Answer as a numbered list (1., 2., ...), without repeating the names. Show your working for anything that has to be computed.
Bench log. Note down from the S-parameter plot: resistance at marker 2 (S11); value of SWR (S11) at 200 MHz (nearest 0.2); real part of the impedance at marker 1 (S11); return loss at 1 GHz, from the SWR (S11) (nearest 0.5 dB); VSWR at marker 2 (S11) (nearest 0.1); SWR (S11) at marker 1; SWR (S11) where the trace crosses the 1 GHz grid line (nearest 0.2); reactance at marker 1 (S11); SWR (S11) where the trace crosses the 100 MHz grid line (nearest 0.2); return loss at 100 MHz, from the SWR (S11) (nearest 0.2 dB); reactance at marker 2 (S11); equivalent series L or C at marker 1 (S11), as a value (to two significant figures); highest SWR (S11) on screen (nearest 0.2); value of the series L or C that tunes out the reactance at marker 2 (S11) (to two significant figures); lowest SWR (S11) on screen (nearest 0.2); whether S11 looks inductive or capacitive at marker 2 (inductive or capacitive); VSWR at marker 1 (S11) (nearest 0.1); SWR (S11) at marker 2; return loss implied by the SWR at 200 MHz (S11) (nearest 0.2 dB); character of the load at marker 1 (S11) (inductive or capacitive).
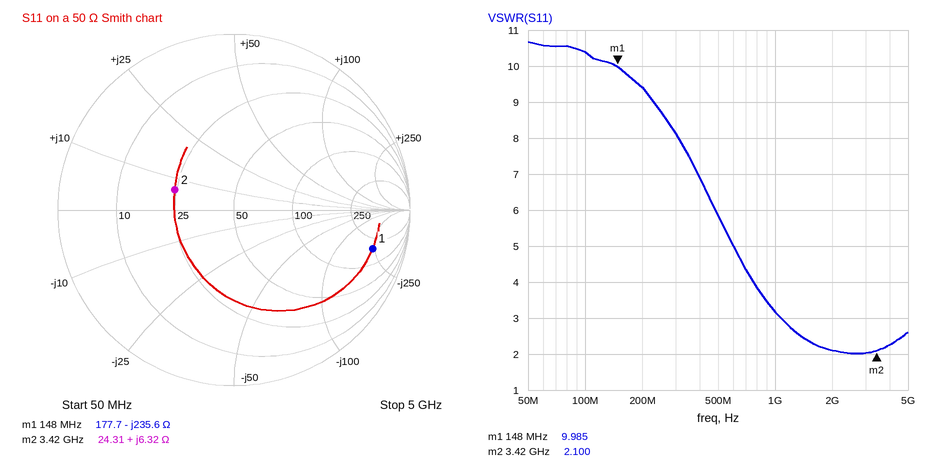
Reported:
1. 24.31 Ω
2. 9.4
3. 177.7 Ω
4. −20 log10((3.2 − 1)/(3.2 + 1)) ≈ 5.62 dB, so 5.5 dB to the nearest 0.5 dB
5. 2.1
6. 9.985
7. 3.2
8. -235.6 Ω
9. 10.4
10. −20 log10((10.4 − 1)/(10.4 + 1)) ≈ 1.68 dB, so 1.6 dB to the nearest 0.2 dB
11. +6.32 Ω
12. C = 1/(2π × 148 MHz × 235.6 Ω) ≈ 4.6 pF
13. 10.6
14. C = 1/(2π × 3.42 GHz × 6.32 Ω) ≈ 7.4 pF
15. 2.0
16. inductive
17. 10.0
18. 2.100
19. −20 log10((9.4 − 1)/(9.4 + 1)) ≈ 1.86 dB, so 1.8 dB to the nearest 0.2 dB
20. capacitive
